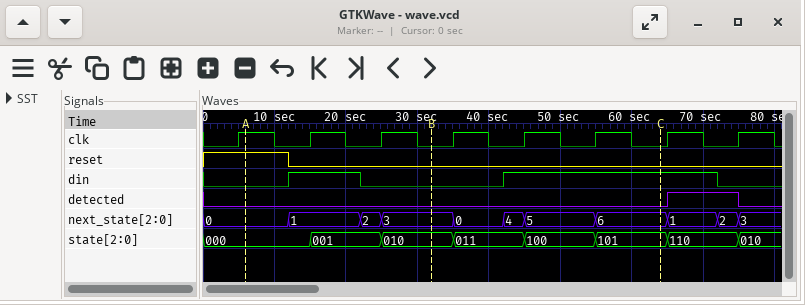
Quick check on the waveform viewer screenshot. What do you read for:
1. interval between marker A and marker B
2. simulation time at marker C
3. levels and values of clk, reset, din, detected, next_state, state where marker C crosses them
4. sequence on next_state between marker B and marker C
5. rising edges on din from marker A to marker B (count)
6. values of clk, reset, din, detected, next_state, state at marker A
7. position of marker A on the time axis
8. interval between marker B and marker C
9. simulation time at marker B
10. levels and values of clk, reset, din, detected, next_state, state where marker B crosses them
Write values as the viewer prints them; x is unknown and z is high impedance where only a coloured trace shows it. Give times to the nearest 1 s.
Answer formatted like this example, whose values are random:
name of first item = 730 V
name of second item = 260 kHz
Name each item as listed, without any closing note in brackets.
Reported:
interval between marker A and marker B = 26 s
simulation time at marker C = 64 s
levels and values of clk, reset, din, detected, next_state, state where marker C crosses them = clk=0, reset=0, din=1, detected=0, next_state=6, state=101
sequence on next_state between marker B and marker C = 3, 0, 4, 5, 6
rising edges on din from marker A to marker B = 1
values of clk, reset, din, detected, next_state, state at marker A = clk=1, reset=1, din=0, detected=0, next_state=0, state=000
position of marker A on the time axis = 6 s
interval between marker B and marker C = 32 s
simulation time at marker B = 32 s
levels and values of clk, reset, din, detected, next_state, state where marker B crosses them = clk=0, reset=0, din=0, detected=0, next_state=3, state=010
